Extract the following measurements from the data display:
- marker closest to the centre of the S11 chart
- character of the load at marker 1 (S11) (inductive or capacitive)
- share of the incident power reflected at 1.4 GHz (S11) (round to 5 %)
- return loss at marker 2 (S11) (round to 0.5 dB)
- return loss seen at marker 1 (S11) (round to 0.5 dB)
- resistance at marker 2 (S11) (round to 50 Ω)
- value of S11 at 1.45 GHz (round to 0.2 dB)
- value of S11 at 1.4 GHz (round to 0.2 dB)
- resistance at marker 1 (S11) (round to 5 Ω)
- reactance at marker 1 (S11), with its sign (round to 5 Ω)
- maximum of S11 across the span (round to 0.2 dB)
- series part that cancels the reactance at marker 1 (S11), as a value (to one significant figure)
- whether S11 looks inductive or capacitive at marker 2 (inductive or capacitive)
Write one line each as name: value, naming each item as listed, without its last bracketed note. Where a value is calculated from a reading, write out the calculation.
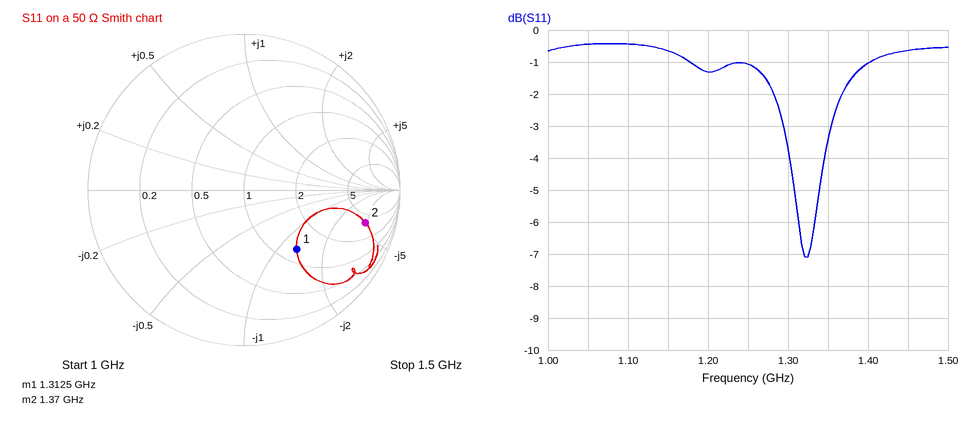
marker closest to the centre of the S11 chart: marker 1
character of the load at marker 1 (S11): capacitive
share of the incident power reflected at 1.4 GHz (S11): 10^(-1/10) ≈ 79.4 %, so 80 % to the nearest 5 %
return loss at marker 2 (S11): 2.0 dB
return loss seen at marker 1 (S11): 6.0 dB
resistance at marker 2 (S11): 200 Ω
value of S11 at 1.45 GHz: -0.6 dB
value of S11 at 1.4 GHz: -1.0 dB
resistance at marker 1 (S11): 65 Ω
reactance at marker 1 (S11), with its sign: -65 Ω
maximum of S11 across the span: -0.4 dB
series part that cancels the reactance at marker 1 (S11), as a value: L = 65 Ω/(2π × 1.3125 GHz) ≈ 8 nH
whether S11 looks inductive or capacitive at marker 2: capacitive
